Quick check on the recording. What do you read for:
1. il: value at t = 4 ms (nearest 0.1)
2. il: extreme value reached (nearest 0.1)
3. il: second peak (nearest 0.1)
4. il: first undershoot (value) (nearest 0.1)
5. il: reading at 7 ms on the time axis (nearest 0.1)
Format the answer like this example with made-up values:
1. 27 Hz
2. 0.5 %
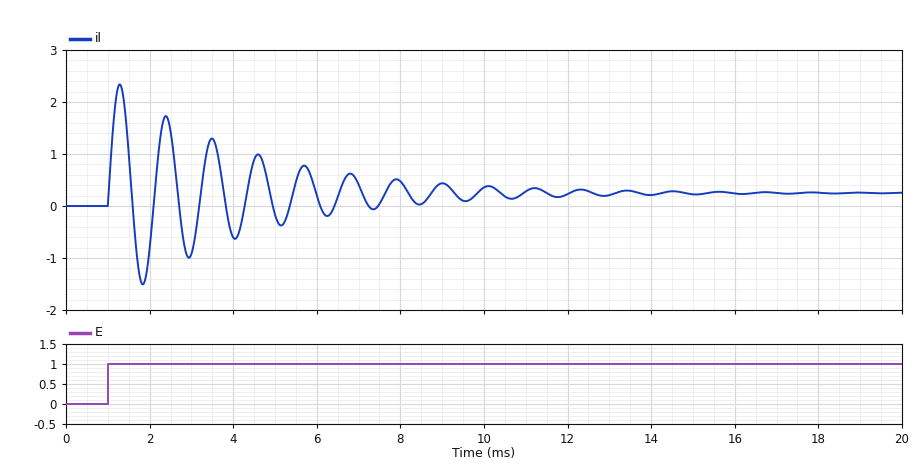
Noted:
1. -0.6
2. 2.3
3. 1.7
4. -1.5
5. 0.4
